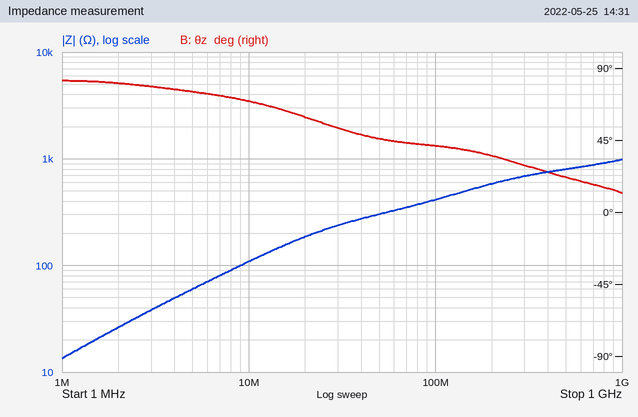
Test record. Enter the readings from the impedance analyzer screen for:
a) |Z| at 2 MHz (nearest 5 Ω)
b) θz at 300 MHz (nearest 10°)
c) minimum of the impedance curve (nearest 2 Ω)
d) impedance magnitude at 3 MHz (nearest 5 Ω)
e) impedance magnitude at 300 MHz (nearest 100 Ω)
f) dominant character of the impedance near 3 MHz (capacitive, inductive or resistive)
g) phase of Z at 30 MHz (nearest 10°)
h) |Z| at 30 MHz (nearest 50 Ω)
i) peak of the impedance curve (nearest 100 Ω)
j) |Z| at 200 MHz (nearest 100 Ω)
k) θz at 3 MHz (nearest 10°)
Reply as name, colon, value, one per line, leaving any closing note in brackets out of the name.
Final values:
|Z| at 2 MHz: 25 Ω
θz at 300 MHz: 30°
minimum of the impedance curve: 14 Ω
impedance magnitude at 3 MHz: 40 Ω
impedance magnitude at 300 MHz: 700 Ω
dominant character of the impedance near 3 MHz: inductive
phase of Z at 30 MHz: 50°
|Z| at 30 MHz: 250 Ω
peak of the impedance curve: 1.0 kΩ
|Z| at 200 MHz: 600 Ω
θz at 3 MHz: 80°
